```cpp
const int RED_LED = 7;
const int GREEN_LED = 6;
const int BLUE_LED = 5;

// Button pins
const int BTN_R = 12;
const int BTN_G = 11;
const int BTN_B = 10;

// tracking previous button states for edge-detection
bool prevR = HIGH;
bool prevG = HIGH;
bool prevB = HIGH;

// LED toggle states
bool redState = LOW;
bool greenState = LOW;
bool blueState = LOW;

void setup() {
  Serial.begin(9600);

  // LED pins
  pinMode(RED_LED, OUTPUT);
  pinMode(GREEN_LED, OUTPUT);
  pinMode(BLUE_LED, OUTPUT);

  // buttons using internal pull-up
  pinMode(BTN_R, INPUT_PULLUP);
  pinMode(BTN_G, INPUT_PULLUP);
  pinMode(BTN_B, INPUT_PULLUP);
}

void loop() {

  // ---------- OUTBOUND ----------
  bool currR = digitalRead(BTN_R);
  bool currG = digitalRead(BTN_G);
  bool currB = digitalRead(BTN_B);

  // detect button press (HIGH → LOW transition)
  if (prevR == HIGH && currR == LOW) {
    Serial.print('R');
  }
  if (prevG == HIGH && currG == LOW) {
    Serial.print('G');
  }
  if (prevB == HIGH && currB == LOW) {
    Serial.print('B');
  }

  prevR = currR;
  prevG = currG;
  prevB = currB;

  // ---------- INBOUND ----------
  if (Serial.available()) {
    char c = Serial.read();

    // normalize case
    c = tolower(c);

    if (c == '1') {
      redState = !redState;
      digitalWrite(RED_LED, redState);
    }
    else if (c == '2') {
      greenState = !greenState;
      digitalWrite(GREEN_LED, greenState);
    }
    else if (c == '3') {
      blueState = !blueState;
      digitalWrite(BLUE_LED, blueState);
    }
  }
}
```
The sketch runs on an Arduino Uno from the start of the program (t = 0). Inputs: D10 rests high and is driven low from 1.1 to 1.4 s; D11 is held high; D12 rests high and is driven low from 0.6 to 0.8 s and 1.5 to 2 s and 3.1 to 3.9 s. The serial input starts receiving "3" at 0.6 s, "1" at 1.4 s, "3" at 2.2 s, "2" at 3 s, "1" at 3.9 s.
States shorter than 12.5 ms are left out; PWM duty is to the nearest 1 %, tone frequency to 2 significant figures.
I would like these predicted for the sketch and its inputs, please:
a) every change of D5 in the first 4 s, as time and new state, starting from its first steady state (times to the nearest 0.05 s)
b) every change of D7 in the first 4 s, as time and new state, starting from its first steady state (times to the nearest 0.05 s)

0 s low; 0.6 s high; 2.2 s low
0 s low; 1.4 s high; 3.9 s low
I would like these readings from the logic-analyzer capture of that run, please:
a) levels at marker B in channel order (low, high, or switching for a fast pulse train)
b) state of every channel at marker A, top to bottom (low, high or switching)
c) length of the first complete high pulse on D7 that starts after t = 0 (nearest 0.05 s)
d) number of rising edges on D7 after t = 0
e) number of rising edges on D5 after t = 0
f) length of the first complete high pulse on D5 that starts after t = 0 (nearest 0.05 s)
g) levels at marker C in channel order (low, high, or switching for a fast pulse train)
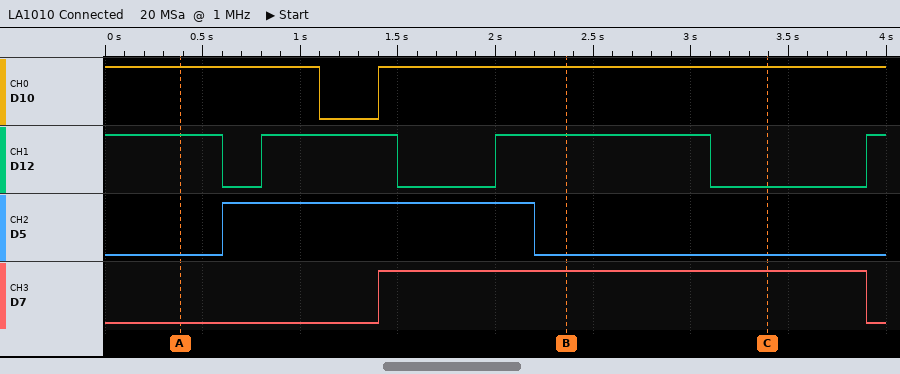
D10 high, D12 high, D5 low, D7 high
D10 high, D12 high, D5 low, D7 low
2.50 s
1
1
1.60 s
D10 high, D12 low, D5 low, D7 high
